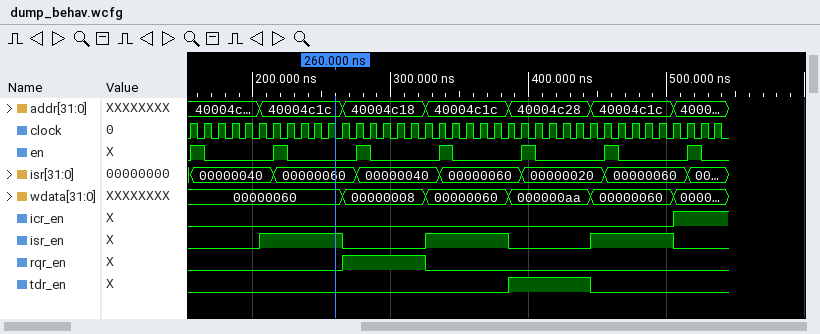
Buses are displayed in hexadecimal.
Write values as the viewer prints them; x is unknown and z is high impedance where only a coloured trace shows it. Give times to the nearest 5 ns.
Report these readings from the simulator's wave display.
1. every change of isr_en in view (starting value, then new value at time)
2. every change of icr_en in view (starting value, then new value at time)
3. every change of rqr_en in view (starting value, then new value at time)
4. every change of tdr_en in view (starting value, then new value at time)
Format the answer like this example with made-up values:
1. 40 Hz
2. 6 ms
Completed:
1. 0, 1 at 205 ns, 0 at 265 ns, 1 at 325 ns, 0 at 385 ns, 1 at 445 ns, 0 at 505 ns
2. 0, 1 at 505 ns
3. 0, 1 at 265 ns, 0 at 325 ns
4. 0, 1 at 385 ns, 0 at 445 ns
